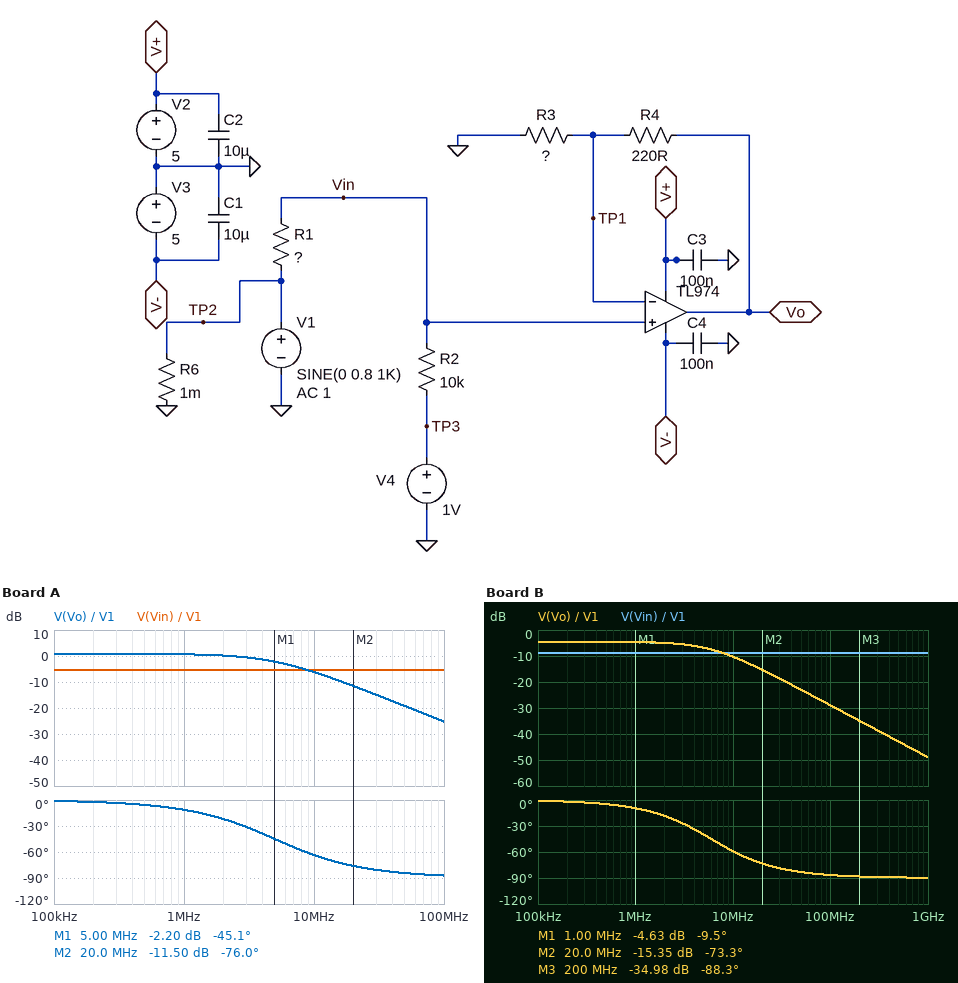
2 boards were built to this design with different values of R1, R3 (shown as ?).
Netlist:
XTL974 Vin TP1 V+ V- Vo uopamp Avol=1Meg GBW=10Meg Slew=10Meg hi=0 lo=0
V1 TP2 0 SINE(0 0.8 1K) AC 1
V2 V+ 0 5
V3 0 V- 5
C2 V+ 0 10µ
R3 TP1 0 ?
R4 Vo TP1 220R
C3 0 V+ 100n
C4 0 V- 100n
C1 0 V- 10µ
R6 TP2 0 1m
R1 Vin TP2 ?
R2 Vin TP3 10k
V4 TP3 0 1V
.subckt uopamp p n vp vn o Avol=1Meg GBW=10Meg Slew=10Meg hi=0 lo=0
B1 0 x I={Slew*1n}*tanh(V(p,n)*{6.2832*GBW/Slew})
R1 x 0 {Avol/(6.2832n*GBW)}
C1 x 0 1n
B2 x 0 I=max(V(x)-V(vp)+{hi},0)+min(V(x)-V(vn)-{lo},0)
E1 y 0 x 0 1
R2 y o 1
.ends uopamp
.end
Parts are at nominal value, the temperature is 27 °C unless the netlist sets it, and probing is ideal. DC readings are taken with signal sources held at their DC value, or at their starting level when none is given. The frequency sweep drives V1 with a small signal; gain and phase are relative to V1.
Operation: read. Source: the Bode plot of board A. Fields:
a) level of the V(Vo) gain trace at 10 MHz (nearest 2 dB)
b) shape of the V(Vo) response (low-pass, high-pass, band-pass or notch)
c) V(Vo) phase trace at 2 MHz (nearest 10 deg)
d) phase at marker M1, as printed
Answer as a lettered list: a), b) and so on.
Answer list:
a) -6 dB
b) low-pass
c) -20 deg
d) -45.1 deg
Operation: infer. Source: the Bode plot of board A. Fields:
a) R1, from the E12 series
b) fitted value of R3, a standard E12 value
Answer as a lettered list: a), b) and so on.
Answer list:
a) 8.2 kΩ
b) 220 Ω
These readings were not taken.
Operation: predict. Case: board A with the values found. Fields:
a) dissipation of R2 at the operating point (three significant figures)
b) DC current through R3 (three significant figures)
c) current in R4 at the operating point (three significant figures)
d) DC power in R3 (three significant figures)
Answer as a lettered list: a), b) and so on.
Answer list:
a) 30.2 µW
b) 2.05 mA
c) 2.05 mA
d) 923 µW
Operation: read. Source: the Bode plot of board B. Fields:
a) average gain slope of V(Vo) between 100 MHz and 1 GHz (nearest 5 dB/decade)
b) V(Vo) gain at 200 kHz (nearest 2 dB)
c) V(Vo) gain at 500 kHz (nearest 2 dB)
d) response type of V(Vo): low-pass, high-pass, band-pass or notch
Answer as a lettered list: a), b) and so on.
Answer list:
a) -20 dB/decade
b) -4 dB
c) -4 dB
d) low-pass
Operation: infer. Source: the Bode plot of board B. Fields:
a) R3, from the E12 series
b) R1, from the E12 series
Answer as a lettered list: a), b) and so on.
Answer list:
a) 330 Ω
b) 18 kΩ
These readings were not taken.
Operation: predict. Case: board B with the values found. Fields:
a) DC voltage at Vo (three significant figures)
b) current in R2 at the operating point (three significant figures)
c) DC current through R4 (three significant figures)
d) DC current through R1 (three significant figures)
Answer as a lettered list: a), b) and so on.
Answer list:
a) 1.07 V
b) 35.7 µA
c) 1.95 mA
d) 35.7 µA
